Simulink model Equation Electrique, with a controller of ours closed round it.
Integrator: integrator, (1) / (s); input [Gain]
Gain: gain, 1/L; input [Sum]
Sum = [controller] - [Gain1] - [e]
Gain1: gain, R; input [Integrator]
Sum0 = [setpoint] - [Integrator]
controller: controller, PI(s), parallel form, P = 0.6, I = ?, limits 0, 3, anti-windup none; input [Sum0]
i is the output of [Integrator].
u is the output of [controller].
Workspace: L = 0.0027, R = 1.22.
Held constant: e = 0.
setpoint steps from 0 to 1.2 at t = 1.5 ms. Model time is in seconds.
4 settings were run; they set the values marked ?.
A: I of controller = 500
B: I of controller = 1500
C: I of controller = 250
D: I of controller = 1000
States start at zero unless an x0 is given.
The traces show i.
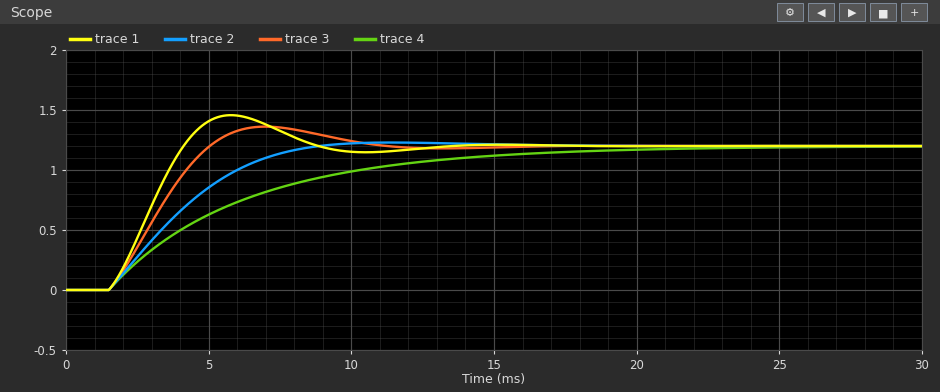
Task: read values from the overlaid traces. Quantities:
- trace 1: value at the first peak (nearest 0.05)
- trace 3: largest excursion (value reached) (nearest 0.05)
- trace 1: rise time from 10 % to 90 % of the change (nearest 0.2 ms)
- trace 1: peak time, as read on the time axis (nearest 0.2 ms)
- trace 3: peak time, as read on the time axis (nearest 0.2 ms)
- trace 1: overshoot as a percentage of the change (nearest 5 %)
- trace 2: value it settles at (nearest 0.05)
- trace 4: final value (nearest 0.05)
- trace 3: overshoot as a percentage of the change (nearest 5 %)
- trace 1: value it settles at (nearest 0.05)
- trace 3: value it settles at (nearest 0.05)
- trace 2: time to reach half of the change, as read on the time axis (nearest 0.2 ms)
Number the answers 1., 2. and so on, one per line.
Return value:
1. 1.45
2. 1.35
3. 2.0 ms
4. 5.8 ms
5. 7.0 ms
6. 20 %
7. 1.20
8. 1.20
9. 15 %
10. 1.20
11. 1.20
12. 3.8 ms
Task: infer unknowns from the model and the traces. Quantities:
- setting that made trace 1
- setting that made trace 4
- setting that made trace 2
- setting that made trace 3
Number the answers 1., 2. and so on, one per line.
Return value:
1. B
2. C
3. A
4. D
